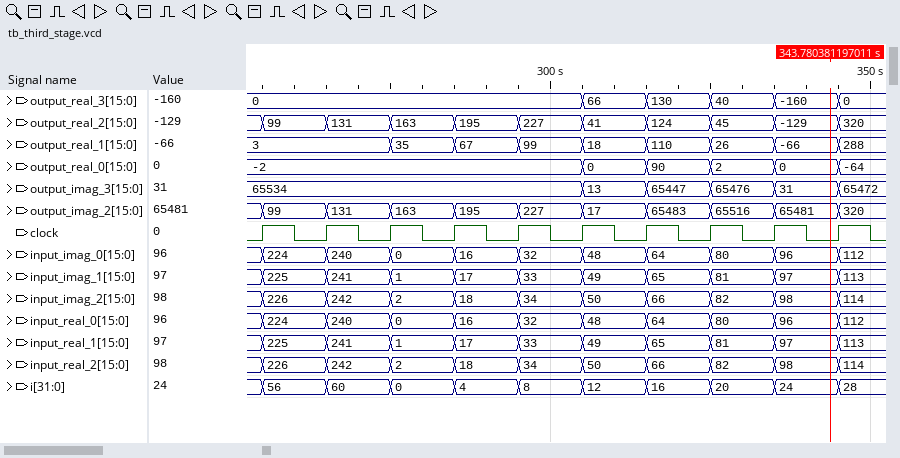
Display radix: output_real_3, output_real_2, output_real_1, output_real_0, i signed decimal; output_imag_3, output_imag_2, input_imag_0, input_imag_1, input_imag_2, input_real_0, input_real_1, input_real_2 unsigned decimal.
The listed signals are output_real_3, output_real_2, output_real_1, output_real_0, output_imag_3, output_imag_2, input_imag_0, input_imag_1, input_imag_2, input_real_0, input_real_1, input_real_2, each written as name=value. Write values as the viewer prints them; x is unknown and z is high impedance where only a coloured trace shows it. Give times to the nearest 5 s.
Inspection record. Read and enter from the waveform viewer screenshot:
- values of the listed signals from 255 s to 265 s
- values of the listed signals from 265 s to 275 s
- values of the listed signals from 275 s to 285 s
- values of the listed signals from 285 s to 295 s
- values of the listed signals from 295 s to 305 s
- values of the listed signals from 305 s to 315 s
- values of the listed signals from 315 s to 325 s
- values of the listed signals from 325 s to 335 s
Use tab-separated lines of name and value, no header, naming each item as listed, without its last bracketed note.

values of the listed signals from 255 s to 265 s	output_real_3=0, output_real_2=99, output_real_1=3, output_real_0=-2, output_imag_3=65534, output_imag_2=99, input_imag_0=224, input_imag_1=225, input_imag_2=226, input_real_0=224, input_real_1=225, input_real_2=226
values of the listed signals from 265 s to 275 s	output_real_3=0, output_real_2=131, output_real_1=3, output_real_0=-2, output_imag_3=65534, output_imag_2=131, input_imag_0=240, input_imag_1=241, input_imag_2=242, input_real_0=240, input_real_1=241, input_real_2=242
values of the listed signals from 275 s to 285 s	output_real_3=0, output_real_2=163, output_real_1=35, output_real_0=-2, output_imag_3=65534, output_imag_2=163, input_imag_0=0, input_imag_1=1, input_imag_2=2, input_real_0=0, input_real_1=1, input_real_2=2
values of the listed signals from 285 s to 295 s	output_real_3=0, output_real_2=195, output_real_1=67, output_real_0=-2, output_imag_3=65534, output_imag_2=195, input_imag_0=16, input_imag_1=17, input_imag_2=18, input_real_0=16, input_real_1=17, input_real_2=18
values of the listed signals from 295 s to 305 s	output_real_3=0, output_real_2=227, output_real_1=99, output_real_0=-2, output_imag_3=65534, output_imag_2=227, input_imag_0=32, input_imag_1=33, input_imag_2=34, input_real_0=32, input_real_1=33, input_real_2=34
values of the listed signals from 305 s to 315 s	output_real_3=66, output_real_2=41, output_real_1=18, output_real_0=0, output_imag_3=13, output_imag_2=17, input_imag_0=48, input_imag_1=49, input_imag_2=50, input_real_0=48, input_real_1=49, input_real_2=50
values of the listed signals from 315 s to 325 s	output_real_3=130, output_real_2=124, output_real_1=110, output_real_0=90, output_imag_3=65447, output_imag_2=65483, input_imag_0=64, input_imag_1=65, input_imag_2=66, input_real_0=64, input_real_1=65, input_real_2=66
values of the listed signals from 325 s to 335 s	output_real_3=40, output_real_2=45, output_real_1=26, output_real_0=2, output_imag_3=65476, output_imag_2=65516, input_imag_0=80, input_imag_1=81, input_imag_2=82, input_real_0=80, input_real_1=81, input_real_2=82
